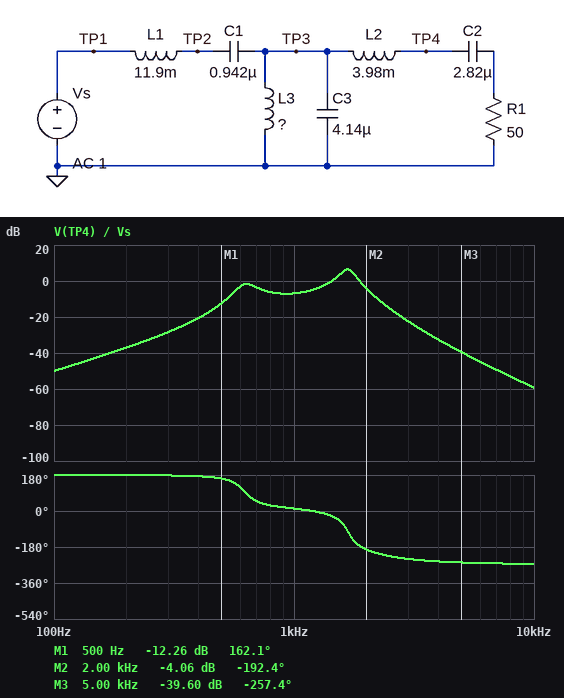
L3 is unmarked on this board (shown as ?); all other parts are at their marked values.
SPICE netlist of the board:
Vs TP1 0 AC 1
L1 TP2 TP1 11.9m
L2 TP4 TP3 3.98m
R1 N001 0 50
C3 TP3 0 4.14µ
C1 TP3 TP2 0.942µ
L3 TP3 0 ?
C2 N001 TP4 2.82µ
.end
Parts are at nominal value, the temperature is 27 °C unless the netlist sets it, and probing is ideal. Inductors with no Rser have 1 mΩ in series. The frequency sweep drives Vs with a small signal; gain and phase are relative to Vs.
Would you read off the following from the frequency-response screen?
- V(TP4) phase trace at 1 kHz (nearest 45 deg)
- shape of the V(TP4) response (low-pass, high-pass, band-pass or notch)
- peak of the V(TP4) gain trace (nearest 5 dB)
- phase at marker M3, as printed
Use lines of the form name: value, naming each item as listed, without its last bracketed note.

V(TP4) phase trace at 1 kHz: 0 deg
shape of the V(TP4) response: band-pass
peak of the V(TP4) gain trace: 5 dB
phase at marker M3, as printed: -257.4 deg
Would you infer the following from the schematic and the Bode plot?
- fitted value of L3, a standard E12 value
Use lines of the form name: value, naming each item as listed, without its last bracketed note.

fitted value of L3, a standard E12 value: 8.2 mH
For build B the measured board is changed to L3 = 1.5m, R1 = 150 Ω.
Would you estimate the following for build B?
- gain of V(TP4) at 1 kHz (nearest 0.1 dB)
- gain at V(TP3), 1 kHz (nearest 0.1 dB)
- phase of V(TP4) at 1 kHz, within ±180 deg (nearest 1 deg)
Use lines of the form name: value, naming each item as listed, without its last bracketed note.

gain of V(TP4) at 1 kHz: -15.8 dB
gain at V(TP3), 1 kHz: -16.2 dB
phase of V(TP4) at 1 kHz, within ±180 deg: 166 deg
